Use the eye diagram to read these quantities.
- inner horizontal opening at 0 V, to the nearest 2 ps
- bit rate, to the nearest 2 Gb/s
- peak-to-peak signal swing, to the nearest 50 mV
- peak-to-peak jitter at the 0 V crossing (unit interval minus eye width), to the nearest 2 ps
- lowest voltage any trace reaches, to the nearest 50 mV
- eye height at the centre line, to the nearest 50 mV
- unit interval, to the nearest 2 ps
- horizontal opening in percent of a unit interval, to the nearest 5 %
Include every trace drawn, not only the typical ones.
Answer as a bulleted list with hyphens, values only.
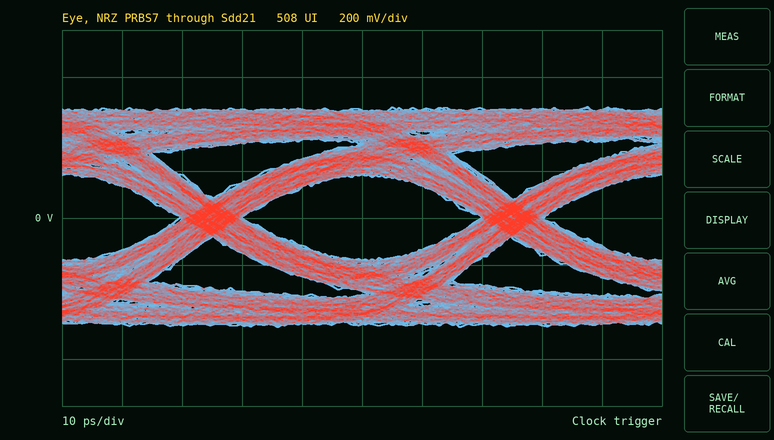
- 40 ps
- 20 Gb/s
- 950 mV
- 10 ps
- -450 mV
- 350 mV
- 50 ps
- 80 %
